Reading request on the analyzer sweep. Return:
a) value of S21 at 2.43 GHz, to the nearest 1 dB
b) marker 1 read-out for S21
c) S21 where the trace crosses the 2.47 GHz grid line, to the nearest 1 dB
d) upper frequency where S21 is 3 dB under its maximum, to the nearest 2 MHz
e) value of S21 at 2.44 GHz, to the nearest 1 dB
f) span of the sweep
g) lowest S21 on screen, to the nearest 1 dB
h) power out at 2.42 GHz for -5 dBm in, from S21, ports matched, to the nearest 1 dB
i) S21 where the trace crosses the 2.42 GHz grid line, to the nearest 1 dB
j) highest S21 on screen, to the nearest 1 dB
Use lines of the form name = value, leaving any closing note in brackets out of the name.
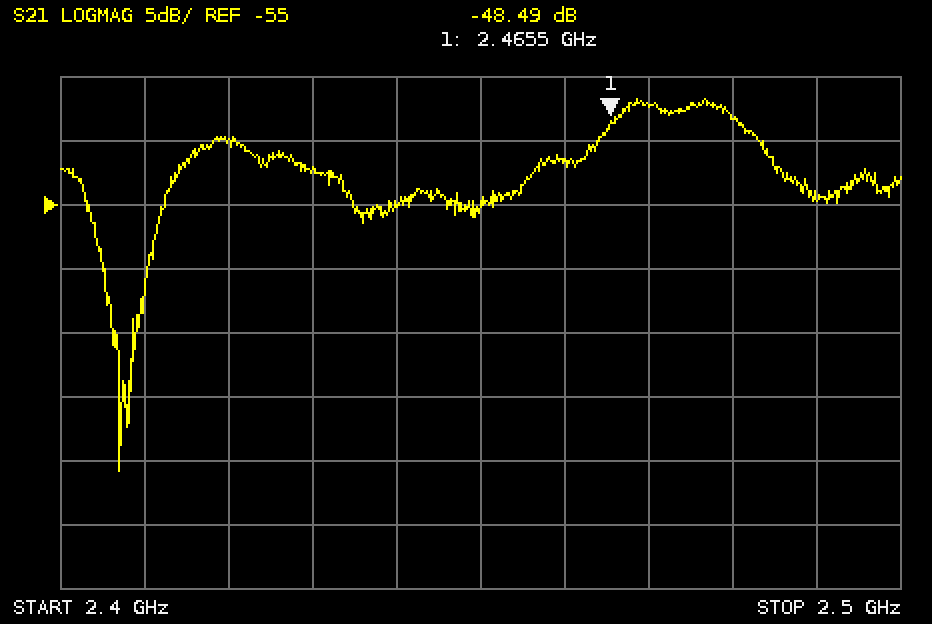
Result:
value of S21 at 2.43 GHz, to the nearest 1 dB = -52 dB
marker 1 read-out for S21 = -48.49 dB
S21 where the trace crosses the 2.47 GHz grid line, to the nearest 1 dB = -47 dB
upper frequency where S21 is 3 dB under its maximum, to the nearest 2 MHz = 2.482 GHz
value of S21 at 2.44 GHz, to the nearest 1 dB = -55 dB
span of the sweep = 100 MHz
lowest S21 on screen, to the nearest 1 dB = -76 dB
power out at 2.42 GHz for -5 dBm in, from S21, ports matched, to the nearest 1 dB = -55 dBm
S21 where the trace crosses the 2.42 GHz grid line, to the nearest 1 dB = -50 dB
highest S21 on screen, to the nearest 1 dB = -47 dB
